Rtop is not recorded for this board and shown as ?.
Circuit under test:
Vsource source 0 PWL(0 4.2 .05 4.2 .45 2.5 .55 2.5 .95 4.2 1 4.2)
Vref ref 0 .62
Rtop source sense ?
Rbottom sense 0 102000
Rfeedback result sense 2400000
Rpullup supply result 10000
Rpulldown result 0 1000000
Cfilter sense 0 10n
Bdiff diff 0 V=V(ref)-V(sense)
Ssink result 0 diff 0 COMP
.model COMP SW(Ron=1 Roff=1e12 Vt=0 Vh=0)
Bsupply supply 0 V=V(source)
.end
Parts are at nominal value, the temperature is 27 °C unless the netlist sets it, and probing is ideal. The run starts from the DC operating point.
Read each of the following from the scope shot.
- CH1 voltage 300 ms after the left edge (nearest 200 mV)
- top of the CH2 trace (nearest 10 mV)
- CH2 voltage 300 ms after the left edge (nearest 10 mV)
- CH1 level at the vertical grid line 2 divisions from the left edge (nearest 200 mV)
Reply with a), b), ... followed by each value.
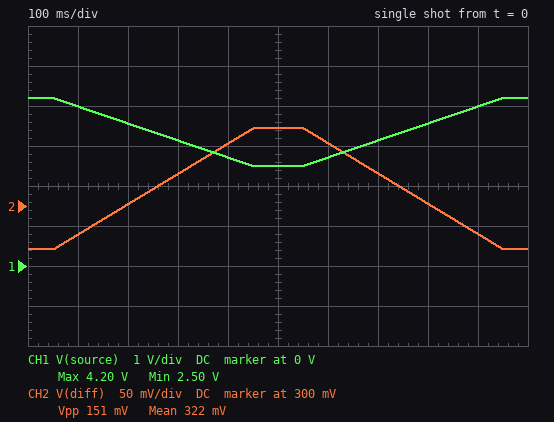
a) 3.2 V
b) 400 mV
c) 340 mV
d) 3.6 V
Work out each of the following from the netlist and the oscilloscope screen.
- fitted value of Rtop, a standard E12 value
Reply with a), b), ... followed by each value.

a) 1 MΩ
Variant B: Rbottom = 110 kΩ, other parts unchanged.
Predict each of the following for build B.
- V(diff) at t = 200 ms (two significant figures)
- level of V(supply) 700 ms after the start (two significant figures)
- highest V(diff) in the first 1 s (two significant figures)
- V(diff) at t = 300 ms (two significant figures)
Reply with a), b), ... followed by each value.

a) 280 mV
b) 3.1 V
c) 380 mV
d) 320 mV
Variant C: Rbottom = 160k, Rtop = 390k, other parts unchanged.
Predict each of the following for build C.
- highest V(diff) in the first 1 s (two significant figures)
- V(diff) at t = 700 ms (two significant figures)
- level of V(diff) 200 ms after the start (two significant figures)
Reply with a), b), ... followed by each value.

a) -190 mV
b) -390 mV
c) -530 mV
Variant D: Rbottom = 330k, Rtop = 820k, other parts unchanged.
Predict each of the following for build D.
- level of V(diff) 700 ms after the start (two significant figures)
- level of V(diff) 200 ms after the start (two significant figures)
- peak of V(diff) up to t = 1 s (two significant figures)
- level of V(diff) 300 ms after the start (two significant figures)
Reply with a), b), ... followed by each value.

a) -470 mV
b) -630 mV
c) -250 mV
d) -480 mV
